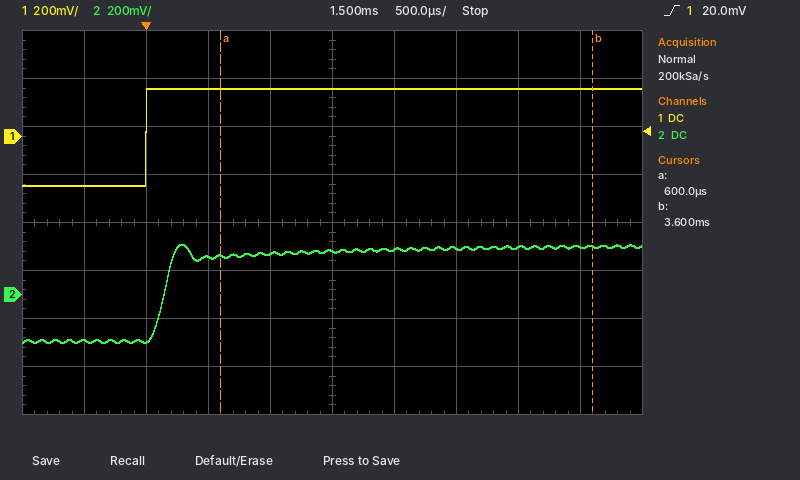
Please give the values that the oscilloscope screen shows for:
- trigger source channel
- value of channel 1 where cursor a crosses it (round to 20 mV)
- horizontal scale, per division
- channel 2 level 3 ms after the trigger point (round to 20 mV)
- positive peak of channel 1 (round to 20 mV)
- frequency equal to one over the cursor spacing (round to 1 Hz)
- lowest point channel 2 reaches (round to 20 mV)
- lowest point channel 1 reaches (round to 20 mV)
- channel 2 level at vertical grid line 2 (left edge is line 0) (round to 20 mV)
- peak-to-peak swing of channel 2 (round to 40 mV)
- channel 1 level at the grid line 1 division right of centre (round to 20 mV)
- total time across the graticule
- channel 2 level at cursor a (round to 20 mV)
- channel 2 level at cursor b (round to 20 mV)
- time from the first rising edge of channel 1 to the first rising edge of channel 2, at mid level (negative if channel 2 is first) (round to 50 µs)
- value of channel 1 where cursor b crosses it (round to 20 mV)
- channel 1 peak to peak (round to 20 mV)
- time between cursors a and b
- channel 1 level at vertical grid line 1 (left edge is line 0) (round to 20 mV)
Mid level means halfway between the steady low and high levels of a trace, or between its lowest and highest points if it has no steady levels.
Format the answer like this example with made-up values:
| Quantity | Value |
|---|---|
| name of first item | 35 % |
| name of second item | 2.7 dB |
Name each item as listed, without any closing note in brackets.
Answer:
| Quantity | Value |
|---|---|
| trigger source channel | channel 1 |
| value of channel 1 where cursor a crosses it | 200 mV |
| horizontal scale, per division | 500 µs |
| channel 2 level 3 ms after the trigger point | 200 mV |
| positive peak of channel 1 | 200 mV |
| frequency equal to one over the cursor spacing | 333 Hz |
| lowest point channel 2 reaches | -200 mV |
| lowest point channel 1 reaches | -200 mV |
| channel 2 level at vertical grid line 2 (left edge is line 0) | -200 mV |
| peak-to-peak swing of channel 2 | 400 mV |
| channel 1 level at the grid line 1 division right of centre | 200 mV |
| total time across the graticule | 5 ms |
| channel 2 level at cursor a | 160 mV |
| channel 2 level at cursor b | 200 mV |
| time from the first rising edge of channel 1 to the first rising edge of channel 2, at mid level (negative if channel 2 is first) | +150 µs |
| value of channel 1 where cursor b crosses it | 200 mV |
| channel 1 peak to peak | 400 mV |
| time between cursors a and b | 3.00 ms |
| channel 1 level at vertical grid line 1 (left edge is line 0) | -200 mV |
